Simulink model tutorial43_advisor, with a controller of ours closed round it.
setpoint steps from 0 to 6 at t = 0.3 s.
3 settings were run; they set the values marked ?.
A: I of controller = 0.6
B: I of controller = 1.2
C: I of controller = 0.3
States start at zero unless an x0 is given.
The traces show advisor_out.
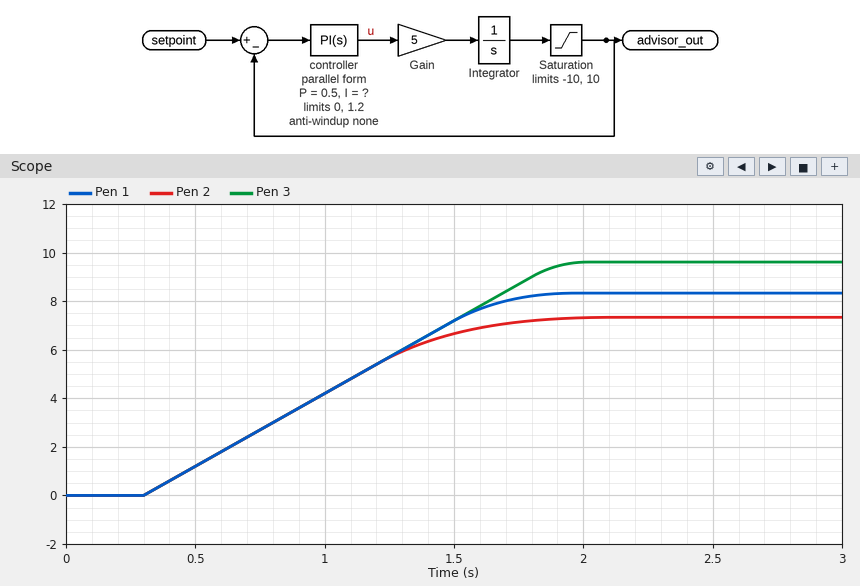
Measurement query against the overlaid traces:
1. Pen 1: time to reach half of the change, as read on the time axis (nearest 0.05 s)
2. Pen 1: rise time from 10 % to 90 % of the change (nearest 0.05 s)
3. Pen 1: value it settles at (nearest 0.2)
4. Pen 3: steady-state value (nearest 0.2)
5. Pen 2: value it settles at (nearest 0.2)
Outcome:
1.00 s
1.10 s
8.4
9.6
7.4
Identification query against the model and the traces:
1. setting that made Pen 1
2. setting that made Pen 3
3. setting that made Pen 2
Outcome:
A
B
C
